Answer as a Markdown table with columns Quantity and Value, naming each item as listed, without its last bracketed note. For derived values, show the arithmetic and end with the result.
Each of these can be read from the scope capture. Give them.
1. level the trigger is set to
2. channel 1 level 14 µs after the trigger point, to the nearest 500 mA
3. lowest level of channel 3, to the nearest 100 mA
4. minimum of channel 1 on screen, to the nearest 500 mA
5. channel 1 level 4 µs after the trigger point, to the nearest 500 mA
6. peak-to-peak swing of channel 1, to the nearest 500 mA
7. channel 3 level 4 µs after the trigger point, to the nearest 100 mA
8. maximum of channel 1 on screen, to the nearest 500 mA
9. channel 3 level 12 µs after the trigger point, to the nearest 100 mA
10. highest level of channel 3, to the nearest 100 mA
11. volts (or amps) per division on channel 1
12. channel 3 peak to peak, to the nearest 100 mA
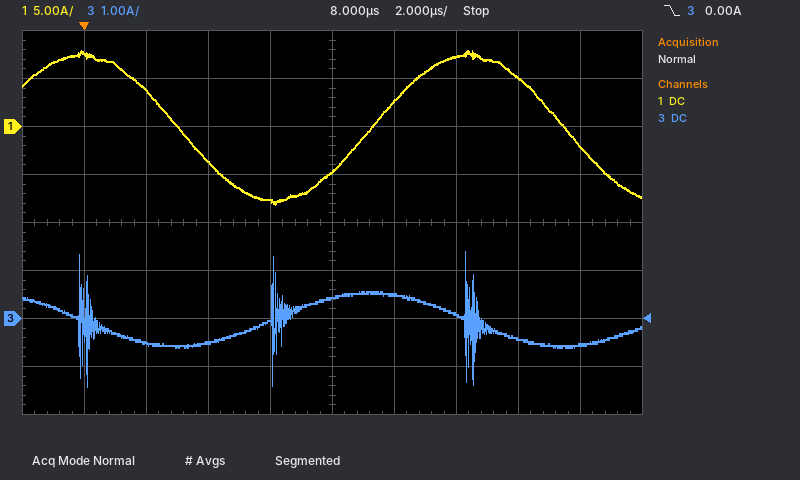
| Quantity | Value |
|---|---|
| level the trigger is set to | 0.00 A |
| channel 1 level 14 µs after the trigger point, to the nearest 500 mA | 5.0 A |
| lowest level of channel 3, to the nearest 100 mA | -1.4 A |
| minimum of channel 1 on screen, to the nearest 500 mA | -8.0 A |
| channel 1 level 4 µs after the trigger point, to the nearest 500 mA | -3.5 A |
| peak-to-peak swing of channel 1, to the nearest 500 mA | 8.0 A − (-8.0 A) = 16.0 A |
| channel 3 level 4 µs after the trigger point, to the nearest 100 mA | -500 mA |
| maximum of channel 1 on screen, to the nearest 500 mA | 8.0 A |
| channel 3 level 12 µs after the trigger point, to the nearest 100 mA | 100 mA |
| highest level of channel 3, to the nearest 100 mA | 1.4 A |
| volts (or amps) per division on channel 1 | 5 A |
| channel 3 peak to peak, to the nearest 100 mA | 1.4 A − (-1.4 A) = 2.8 A |
